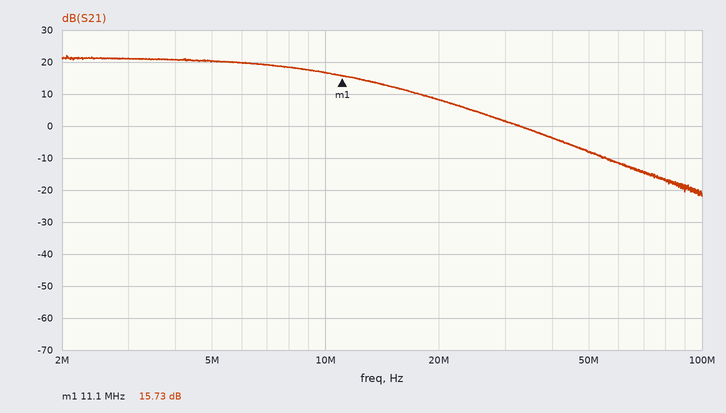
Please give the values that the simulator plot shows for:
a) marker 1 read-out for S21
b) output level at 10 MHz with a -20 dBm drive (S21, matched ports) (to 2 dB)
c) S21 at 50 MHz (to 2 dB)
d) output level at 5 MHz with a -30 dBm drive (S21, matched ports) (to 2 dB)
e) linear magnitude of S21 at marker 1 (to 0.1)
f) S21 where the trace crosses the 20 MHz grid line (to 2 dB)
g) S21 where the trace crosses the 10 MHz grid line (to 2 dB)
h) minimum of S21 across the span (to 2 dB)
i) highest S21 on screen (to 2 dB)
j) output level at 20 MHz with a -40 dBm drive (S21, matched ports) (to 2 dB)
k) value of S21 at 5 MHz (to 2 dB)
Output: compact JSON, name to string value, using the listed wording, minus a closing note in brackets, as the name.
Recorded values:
{"marker 1 read-out for S21": "15.73 dB", "output level at 10 MHz with a -20 dBm drive (S21, matched ports)": "-4 dBm", "S21 at 50 MHz": "-8 dB", "output level at 5 MHz with a -30 dBm drive (S21, matched ports)": "-10 dBm", "linear magnitude of S21 at marker 1": "6.1", "S21 where the trace crosses the 20 MHz grid line": "8 dB", "S21 where the trace crosses the 10 MHz grid line": "16 dB", "minimum of S21 across the span": "-22 dB", "highest S21 on screen": "22 dB", "output level at 20 MHz with a -40 dBm drive (S21, matched ports)": "-32 dBm", "value of S21 at 5 MHz": "20 dB"}
